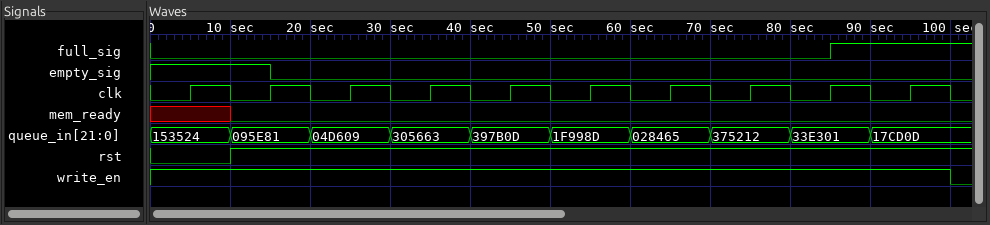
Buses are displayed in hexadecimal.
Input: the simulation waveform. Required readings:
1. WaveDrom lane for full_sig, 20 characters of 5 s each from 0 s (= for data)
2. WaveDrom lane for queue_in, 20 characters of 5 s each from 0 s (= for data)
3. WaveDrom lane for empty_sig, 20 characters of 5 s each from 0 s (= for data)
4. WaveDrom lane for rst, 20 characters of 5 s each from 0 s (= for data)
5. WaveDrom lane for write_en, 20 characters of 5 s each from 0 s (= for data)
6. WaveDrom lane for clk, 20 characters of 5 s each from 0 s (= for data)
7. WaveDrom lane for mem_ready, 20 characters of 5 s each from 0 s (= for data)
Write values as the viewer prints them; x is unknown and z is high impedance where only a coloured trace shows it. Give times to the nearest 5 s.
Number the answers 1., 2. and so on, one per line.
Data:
1. {name: 'full_sig', wave: '0................1..'}
2. {name: 'queue_in', wave: '=.=.=.=.=.=.=.=.=.=.', data: '153524 095E81 04D609 305663 397B0D 1F998D 028465 375212 33E301 17CD0D'}
3. {name: 'empty_sig', wave: '1..0................'}
4. {name: 'rst', wave: '0.1.................'}
5. {name: 'write_en', wave: '1...................'}
6. {name: 'clk', wave: '01010101010101010101'}
7. {name: 'mem_ready', wave: 'x.0.................'}
